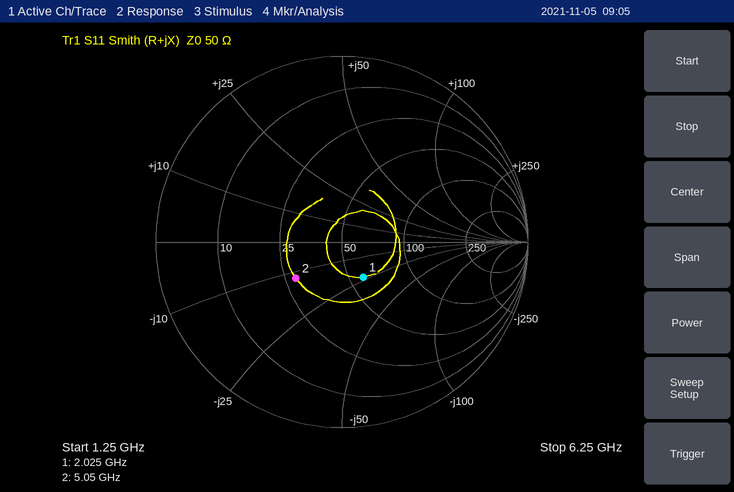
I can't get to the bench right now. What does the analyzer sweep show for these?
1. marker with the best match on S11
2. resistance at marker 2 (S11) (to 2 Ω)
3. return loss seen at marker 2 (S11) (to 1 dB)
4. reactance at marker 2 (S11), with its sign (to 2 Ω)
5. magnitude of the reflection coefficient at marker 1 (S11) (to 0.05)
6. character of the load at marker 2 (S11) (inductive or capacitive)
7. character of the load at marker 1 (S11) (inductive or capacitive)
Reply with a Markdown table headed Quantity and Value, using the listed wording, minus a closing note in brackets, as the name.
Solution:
| Quantity | Value |
|---|---|
| marker with the best match on S11 | marker 1 |
| resistance at marker 2 (S11) | 28 Ω |
| return loss seen at marker 2 (S11) | 10 dB |
| reactance at marker 2 (S11), with its sign | -12 Ω |
| magnitude of the reflection coefficient at marker 1 (S11) | 0.20 |
| character of the load at marker 2 (S11) | capacitive |
| character of the load at marker 1 (S11) | capacitive |
